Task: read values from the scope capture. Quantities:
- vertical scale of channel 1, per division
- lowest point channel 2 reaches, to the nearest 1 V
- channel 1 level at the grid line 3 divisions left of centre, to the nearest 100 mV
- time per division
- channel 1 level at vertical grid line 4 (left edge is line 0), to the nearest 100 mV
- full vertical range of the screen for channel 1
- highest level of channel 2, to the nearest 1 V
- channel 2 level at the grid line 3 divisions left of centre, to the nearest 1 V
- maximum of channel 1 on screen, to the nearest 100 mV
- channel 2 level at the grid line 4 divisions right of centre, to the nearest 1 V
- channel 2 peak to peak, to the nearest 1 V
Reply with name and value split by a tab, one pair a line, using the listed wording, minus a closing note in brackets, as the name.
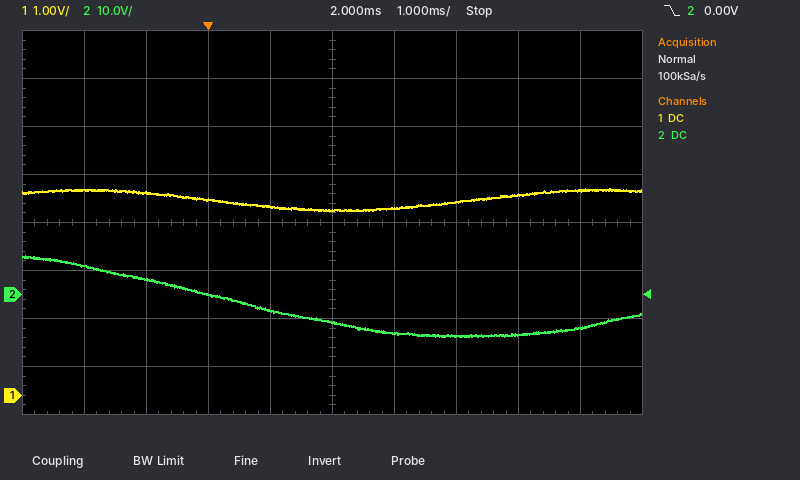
vertical scale of channel 1, per division	1 V
lowest point channel 2 reaches, to the nearest 1 V	-9 V
channel 1 level at the grid line 3 divisions left of centre, to the nearest 100 mV	4.2 V
time per division	1 ms
channel 1 level at vertical grid line 4 (left edge is line 0), to the nearest 100 mV	3.9 V
full vertical range of the screen for channel 1	8 V
highest level of channel 2, to the nearest 1 V	8 V
channel 2 level at the grid line 3 divisions left of centre, to the nearest 1 V	3 V
maximum of channel 1 on screen, to the nearest 100 mV	4.3 V
channel 2 level at the grid line 4 divisions right of centre, to the nearest 1 V	-7 V
channel 2 peak to peak, to the nearest 1 V	17 V
